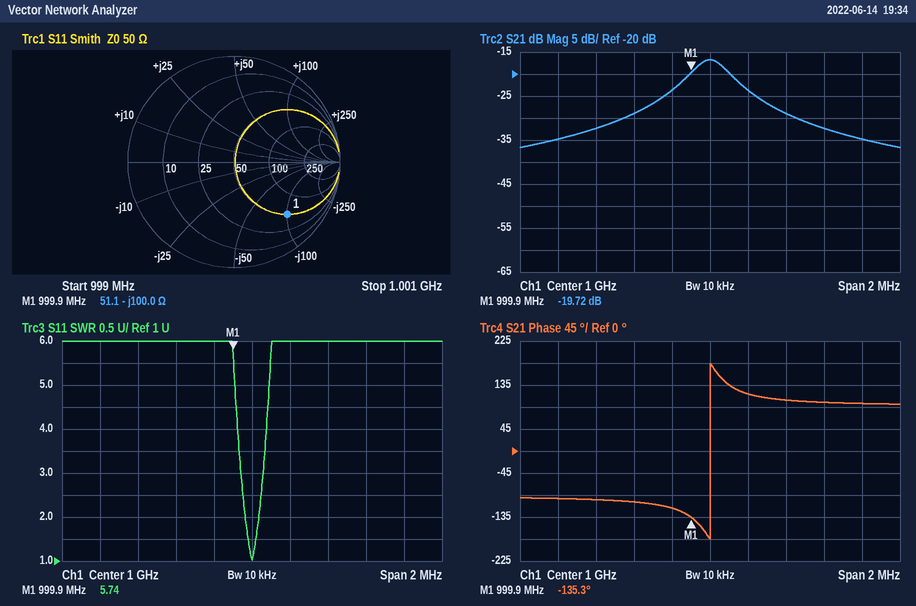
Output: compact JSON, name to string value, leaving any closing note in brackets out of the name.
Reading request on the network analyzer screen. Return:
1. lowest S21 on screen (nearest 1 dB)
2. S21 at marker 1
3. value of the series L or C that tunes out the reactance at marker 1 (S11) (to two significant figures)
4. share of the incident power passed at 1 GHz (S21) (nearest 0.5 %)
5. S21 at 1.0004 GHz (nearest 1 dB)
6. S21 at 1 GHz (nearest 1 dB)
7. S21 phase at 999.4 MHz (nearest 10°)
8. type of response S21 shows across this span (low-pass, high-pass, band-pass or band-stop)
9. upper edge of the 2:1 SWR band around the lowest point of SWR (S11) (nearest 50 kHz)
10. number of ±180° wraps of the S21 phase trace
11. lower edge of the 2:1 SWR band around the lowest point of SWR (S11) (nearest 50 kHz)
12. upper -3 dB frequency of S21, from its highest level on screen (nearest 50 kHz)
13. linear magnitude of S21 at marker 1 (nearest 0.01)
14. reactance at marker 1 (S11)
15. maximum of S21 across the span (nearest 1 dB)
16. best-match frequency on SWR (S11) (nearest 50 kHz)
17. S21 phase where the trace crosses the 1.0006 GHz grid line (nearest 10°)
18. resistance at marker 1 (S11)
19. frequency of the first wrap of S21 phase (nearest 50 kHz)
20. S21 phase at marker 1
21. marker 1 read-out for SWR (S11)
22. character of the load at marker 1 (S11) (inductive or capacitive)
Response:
{"lowest S21 on screen": "-37 dB", "S21 at marker 1": "-19.72 dB", "value of the series L or C that tunes out the reactance at marker 1 (S11)": "16 nH", "share of the incident power passed at 1 GHz (S21)": "2.0 %", "S21 at 1.0004 GHz": "-29 dB", "S21 at 1 GHz": "-17 dB", "S21 phase at 999.4 MHz": "-100°", "type of response S21 shows across this span": "band-pass", "upper edge of the 2:1 SWR band around the lowest point of SWR (S11)": "1.00005 GHz", "number of ±180° wraps of the S21 phase trace": "1", "lower edge of the 2:1 SWR band around the lowest point of SWR (S11)": "999.95 MHz", "upper -3 dB frequency of S21, from its highest level on screen": "1.00010 GHz", "linear magnitude of S21 at marker 1": "0.10", "reactance at marker 1": "-100.0 Ω", "maximum of S21 across the span": "-17 dB", "best-match frequency on SWR (S11)": "1.00000 GHz", "S21 phase where the trace crosses the 1.0006 GHz grid line": "100°", "resistance at marker 1": "51.1 Ω", "frequency of the first wrap of S21 phase": "1.00000 GHz", "S21 phase at marker 1": "-135.3°", "marker 1 read-out for SWR": "5.74", "character of the load at marker 1 (S11)": "capacitive"}
